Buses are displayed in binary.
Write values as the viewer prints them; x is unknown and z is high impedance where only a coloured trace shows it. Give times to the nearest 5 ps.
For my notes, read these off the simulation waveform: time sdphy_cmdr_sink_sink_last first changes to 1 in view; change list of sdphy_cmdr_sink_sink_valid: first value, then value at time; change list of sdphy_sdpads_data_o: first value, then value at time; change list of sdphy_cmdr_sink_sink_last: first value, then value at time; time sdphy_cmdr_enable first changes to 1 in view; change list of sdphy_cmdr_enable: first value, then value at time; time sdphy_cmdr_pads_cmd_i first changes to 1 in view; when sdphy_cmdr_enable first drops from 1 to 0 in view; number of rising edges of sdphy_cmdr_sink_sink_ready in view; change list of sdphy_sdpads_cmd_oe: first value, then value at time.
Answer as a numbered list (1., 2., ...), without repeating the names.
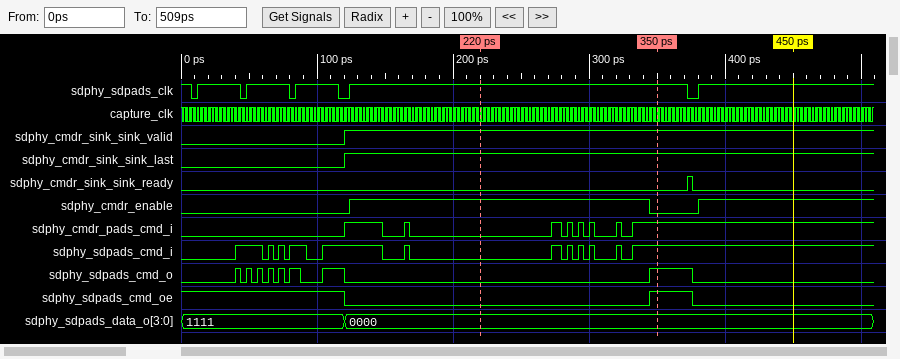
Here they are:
1. 120 ps
2. 0, 1 at 120 ps
3. 1111, 0000 at 120 ps
4. 0, 1 at 120 ps
5. 125 ps
6. 0, 1 at 125 ps, 0 at 345 ps, 1 at 380 ps
7. 120 ps
8. 345 ps
9. 1
10. 1, 0 at 120 ps, 1 at 345 ps, 0 at 375 ps
